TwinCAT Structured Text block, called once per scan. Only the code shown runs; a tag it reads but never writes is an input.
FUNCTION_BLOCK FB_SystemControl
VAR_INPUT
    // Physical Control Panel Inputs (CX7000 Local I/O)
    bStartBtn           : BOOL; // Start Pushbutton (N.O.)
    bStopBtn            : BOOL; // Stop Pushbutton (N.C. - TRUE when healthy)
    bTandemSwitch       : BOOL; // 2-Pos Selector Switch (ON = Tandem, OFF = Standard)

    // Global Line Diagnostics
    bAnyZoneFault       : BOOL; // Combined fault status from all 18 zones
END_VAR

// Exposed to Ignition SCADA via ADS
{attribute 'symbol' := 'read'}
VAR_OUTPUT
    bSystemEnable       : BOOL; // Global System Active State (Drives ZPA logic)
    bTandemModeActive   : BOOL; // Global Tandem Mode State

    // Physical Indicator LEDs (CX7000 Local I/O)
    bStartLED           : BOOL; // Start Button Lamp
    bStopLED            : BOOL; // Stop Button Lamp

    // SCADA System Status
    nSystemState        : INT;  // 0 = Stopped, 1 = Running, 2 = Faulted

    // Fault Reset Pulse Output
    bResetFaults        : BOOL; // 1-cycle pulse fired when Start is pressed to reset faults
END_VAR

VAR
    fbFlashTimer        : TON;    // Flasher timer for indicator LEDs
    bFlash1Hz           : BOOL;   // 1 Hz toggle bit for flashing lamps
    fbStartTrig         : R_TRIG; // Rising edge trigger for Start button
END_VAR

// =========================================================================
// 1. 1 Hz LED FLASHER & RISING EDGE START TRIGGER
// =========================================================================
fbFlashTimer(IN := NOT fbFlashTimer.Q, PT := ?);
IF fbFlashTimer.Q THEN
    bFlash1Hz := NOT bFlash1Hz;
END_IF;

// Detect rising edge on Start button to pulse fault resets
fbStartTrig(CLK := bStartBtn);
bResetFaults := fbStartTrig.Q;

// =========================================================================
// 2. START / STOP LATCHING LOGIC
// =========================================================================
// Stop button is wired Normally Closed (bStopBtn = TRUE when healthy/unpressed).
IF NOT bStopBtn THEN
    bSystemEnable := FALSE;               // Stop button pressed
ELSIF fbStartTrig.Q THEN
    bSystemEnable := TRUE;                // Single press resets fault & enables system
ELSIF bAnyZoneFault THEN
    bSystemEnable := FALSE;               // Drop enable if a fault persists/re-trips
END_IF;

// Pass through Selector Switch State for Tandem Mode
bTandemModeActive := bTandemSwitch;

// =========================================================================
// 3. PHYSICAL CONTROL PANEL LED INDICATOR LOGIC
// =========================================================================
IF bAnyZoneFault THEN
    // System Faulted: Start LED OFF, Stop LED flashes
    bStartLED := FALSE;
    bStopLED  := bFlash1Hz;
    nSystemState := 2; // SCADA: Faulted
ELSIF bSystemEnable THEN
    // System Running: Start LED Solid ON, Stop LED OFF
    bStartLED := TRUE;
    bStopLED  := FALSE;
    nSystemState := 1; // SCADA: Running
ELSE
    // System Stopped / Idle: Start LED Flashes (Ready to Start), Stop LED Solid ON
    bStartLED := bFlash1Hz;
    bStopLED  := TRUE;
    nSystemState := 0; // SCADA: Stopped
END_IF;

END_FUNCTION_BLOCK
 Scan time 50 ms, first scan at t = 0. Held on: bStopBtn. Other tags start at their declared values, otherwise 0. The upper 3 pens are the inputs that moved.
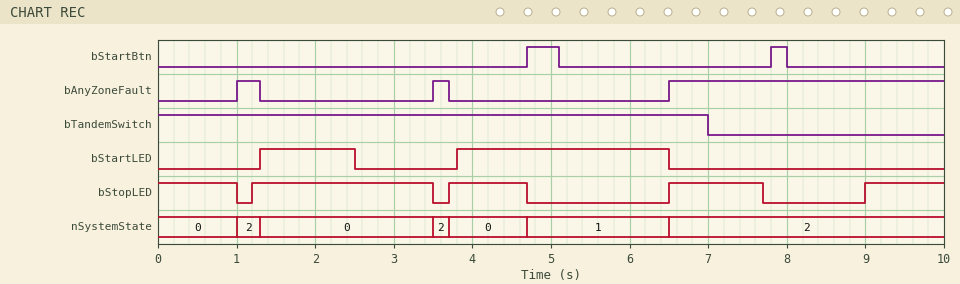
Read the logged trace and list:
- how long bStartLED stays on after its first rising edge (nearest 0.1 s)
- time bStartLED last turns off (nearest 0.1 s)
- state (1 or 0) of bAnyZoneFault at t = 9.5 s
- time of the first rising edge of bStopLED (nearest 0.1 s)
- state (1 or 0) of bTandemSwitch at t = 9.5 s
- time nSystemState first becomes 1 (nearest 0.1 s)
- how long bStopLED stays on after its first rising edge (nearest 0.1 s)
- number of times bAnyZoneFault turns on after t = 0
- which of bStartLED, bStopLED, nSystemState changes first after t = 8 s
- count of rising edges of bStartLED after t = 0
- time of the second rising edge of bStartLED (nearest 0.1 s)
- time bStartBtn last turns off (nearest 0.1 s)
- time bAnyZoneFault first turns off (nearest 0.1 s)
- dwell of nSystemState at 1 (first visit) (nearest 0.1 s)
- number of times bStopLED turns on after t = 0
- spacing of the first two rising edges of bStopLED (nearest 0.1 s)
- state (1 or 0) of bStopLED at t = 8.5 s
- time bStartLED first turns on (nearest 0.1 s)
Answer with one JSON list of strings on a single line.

["1.2 s", "6.5 s", "1", "1.2 s", "0", "4.7 s", "2.3 s", "3", "bStopLED", "2", "3.8 s", "8.0 s", "1.3 s", "1.8 s", "4", "2.5 s", "0", "1.3 s"]
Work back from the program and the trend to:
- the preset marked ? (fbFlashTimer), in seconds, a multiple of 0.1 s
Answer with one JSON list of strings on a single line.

["1.2 s"]
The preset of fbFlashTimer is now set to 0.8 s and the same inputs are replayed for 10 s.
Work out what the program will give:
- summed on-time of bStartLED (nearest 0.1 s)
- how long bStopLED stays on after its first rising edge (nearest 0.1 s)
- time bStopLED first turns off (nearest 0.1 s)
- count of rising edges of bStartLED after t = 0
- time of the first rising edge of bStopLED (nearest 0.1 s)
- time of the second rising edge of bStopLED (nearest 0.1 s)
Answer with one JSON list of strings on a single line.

["3.6 s", "1.0 s", "3.5 s", "4", "3.7 s", "6.5 s"]
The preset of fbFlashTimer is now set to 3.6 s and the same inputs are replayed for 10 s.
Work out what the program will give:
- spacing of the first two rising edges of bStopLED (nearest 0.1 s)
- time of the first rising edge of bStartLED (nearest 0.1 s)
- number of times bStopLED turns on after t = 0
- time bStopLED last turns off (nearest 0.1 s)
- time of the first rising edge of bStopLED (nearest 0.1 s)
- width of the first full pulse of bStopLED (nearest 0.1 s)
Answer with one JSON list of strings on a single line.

["2.3 s", "3.7 s", "3", "7.3 s", "1.3 s", "2.2 s"]
